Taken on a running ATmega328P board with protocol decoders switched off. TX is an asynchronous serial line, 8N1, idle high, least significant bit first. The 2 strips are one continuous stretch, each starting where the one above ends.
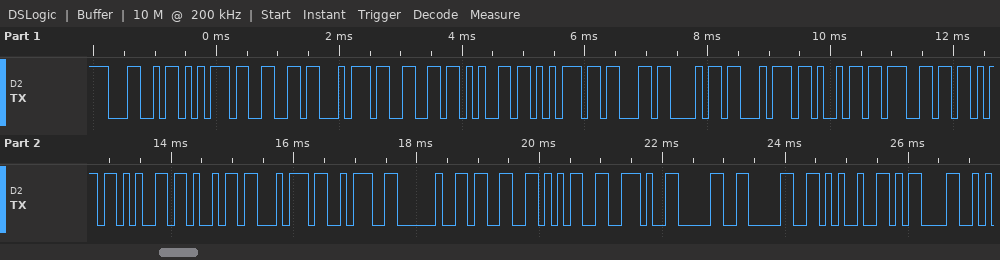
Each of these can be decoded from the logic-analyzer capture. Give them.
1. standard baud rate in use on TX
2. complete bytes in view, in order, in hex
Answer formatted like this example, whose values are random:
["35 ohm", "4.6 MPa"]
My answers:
["9600 baud", "4C 75 66 74 66 65 75 63 68 74 69 67 6B 65 69 74 3A 20 33 35 2E 30 30 25 0D"]
